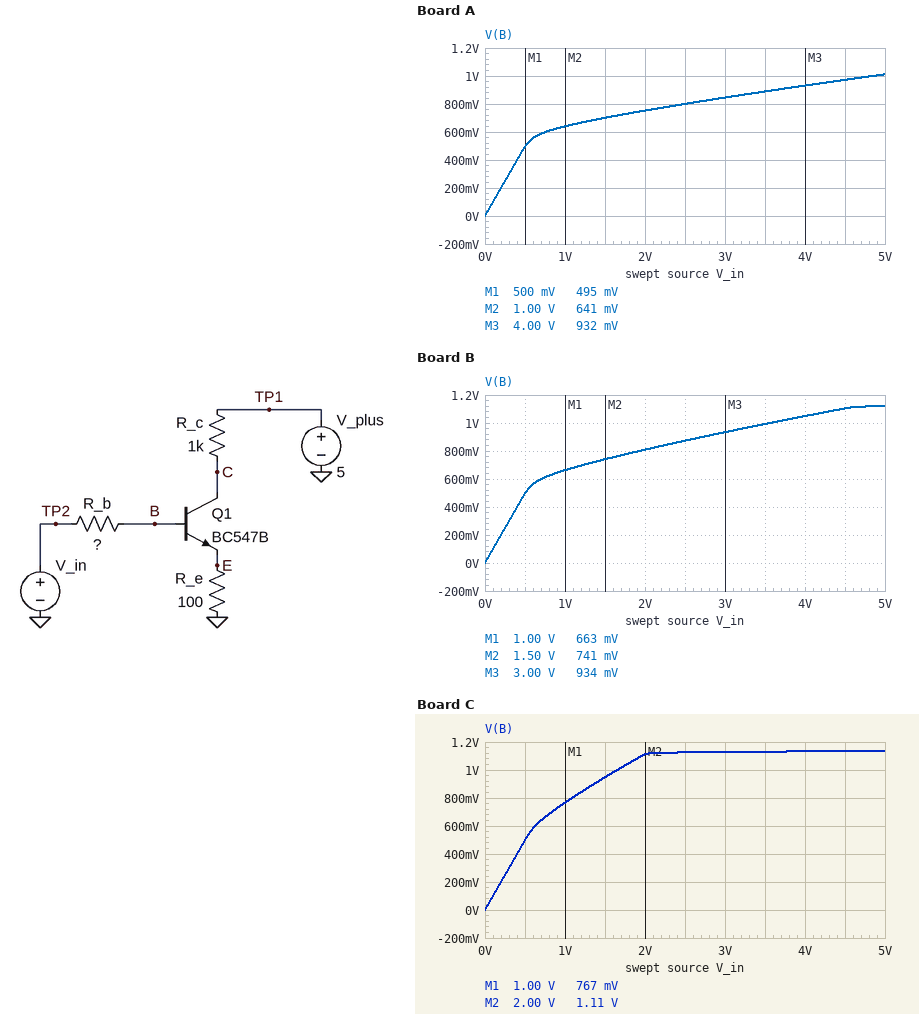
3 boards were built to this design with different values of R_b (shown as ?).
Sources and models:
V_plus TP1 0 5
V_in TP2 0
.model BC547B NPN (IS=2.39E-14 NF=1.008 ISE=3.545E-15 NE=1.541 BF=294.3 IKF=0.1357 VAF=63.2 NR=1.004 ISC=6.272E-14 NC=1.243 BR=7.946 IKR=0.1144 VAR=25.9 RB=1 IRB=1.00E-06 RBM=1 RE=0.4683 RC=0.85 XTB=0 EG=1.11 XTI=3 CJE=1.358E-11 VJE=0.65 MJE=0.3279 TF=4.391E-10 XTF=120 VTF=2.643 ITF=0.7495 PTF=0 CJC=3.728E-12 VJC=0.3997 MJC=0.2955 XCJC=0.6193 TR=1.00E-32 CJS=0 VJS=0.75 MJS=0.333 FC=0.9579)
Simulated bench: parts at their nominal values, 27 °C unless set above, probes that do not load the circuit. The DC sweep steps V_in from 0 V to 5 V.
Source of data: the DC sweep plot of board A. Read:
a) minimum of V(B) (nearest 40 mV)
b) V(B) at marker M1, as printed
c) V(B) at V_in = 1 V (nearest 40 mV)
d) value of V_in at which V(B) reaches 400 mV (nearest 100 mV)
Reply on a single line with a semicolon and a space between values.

0 V; 495 mV; 640 mV; 400 mV
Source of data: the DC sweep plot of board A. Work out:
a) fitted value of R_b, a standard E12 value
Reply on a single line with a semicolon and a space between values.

330 kΩ
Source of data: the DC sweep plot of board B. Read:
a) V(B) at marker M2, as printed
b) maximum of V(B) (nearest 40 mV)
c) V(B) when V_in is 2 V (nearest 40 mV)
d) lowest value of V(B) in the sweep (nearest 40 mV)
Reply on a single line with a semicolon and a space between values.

741 mV; 1.12 V; 800 mV; 0 V
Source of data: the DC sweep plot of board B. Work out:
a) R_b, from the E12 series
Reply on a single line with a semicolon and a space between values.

220 kΩ
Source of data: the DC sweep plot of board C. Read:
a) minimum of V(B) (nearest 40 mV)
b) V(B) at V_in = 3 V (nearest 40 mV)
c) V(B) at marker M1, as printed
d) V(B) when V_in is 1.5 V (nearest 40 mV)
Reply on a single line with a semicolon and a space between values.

0 V; 1.12 V; 767 mV; 960 mV
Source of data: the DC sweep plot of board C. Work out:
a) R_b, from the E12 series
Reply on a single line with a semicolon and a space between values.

56 kΩ
